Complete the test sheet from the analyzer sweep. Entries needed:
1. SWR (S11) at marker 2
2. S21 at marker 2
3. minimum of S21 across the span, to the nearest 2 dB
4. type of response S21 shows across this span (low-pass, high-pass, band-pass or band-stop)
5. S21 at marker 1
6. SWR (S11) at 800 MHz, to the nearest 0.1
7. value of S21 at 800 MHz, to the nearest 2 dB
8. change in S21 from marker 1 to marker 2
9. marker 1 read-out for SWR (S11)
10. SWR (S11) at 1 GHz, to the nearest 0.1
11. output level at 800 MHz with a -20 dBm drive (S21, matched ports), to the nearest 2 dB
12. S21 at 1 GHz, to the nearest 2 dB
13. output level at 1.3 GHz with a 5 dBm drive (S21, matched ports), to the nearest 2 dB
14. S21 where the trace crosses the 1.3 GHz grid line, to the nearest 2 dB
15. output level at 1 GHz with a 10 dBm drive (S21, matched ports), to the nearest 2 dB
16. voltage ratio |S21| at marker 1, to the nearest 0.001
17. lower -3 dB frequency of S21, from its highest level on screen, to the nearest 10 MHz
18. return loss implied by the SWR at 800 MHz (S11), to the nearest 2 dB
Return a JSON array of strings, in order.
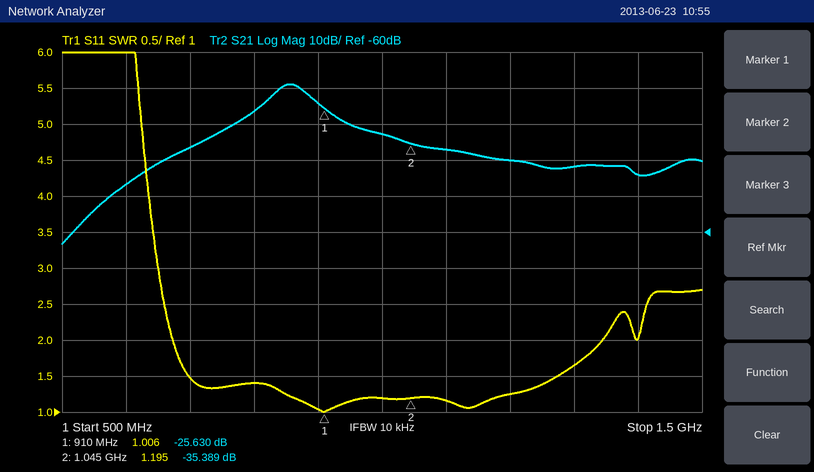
["1.195", "-35.389 dB", "-64 dB", "band-pass", "-25.630 dB", "1.4", "-26 dB", "-9.759 dB", "1.006", "1.2", "-46 dBm", "-32 dB", "-36 dBm", "-42 dB", "-22 dBm", "0.052", "830 MHz", "16 dB"]
